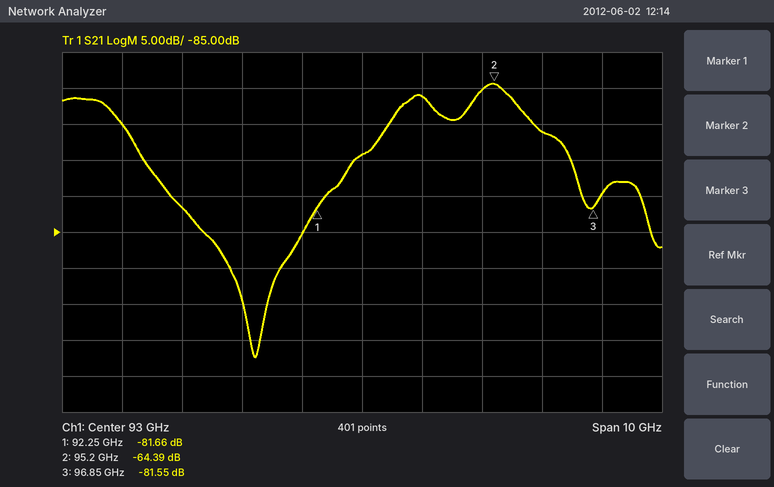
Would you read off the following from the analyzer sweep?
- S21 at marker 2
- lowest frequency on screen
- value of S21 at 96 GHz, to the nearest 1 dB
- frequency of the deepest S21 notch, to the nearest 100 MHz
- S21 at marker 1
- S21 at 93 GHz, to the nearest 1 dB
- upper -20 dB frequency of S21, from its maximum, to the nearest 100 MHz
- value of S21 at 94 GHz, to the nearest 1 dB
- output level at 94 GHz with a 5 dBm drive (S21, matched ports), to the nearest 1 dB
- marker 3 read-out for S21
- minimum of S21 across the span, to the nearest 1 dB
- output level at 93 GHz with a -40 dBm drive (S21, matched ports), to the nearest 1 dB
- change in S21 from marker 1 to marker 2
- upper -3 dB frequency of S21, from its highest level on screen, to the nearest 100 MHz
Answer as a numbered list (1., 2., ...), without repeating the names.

1. -64.39 dB
2. 88 GHz
3. -71 dB
4. 91.2 GHz
5. -81.66 dB
6. -74 dB
7. 97.8 GHz
8. -66 dB
9. -61 dBm
10. -81.55 dB
11. -102 dB
12. -114 dBm
13. 17.27 dB
14. 95.6 GHz
